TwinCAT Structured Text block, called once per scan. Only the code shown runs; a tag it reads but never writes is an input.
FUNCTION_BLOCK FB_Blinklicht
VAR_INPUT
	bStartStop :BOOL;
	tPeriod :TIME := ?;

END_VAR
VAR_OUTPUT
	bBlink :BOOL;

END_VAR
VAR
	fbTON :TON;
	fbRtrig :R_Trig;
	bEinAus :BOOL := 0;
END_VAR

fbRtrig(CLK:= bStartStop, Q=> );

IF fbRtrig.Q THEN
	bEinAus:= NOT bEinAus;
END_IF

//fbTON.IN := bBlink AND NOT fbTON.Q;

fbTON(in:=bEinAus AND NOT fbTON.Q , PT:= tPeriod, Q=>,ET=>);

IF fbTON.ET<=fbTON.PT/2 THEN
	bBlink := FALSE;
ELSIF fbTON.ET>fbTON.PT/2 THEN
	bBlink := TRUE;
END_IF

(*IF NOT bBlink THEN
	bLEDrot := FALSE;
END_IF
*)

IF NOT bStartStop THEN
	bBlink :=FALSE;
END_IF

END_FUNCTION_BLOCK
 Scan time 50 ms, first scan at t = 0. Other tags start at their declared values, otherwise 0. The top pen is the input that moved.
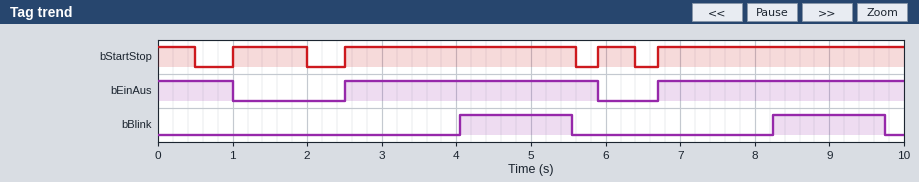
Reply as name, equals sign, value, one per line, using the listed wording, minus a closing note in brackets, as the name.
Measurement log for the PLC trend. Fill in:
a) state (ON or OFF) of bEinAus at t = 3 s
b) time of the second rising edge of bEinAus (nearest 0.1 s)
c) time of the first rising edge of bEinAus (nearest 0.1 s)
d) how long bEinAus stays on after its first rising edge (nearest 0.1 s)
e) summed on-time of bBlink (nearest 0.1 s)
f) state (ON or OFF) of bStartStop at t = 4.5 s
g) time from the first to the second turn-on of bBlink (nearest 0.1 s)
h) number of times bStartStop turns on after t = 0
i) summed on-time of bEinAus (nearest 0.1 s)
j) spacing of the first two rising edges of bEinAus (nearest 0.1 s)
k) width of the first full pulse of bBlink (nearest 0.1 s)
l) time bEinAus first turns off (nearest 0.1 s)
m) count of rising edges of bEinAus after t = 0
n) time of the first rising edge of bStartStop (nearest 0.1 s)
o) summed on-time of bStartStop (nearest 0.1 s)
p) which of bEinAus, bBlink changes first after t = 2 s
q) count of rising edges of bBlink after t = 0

state (ON or OFF) of bEinAus at t = 3 s = ON
time of the second rising edge of bEinAus = 6.7 s
time of the first rising edge of bEinAus = 2.5 s
how long bEinAus stays on after its first rising edge = 3.4 s
summed on-time of bBlink = 3.0 s
state (ON or OFF) of bStartStop at t = 4.5 s = ON
time from the first to the second turn-on of bBlink = 4.2 s
number of times bStartStop turns on after t = 0 = 4
summed on-time of bEinAus = 7.7 s
spacing of the first two rising edges of bEinAus = 4.2 s
width of the first full pulse of bBlink = 1.5 s
time bEinAus first turns off = 1.0 s
count of rising edges of bEinAus after t = 0 = 2
time of the first rising edge of bStartStop = 1.0 s
summed on-time of bStartStop = 8.4 s
which of bEinAus, bBlink changes first after t = 2 s = bEinAus
count of rising edges of bBlink after t = 0 = 2
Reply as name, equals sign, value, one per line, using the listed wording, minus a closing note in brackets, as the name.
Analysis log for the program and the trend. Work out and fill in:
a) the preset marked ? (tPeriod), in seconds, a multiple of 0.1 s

the preset marked ? (tPeriod), in seconds, a multiple of 0.1 s = 3.0 s
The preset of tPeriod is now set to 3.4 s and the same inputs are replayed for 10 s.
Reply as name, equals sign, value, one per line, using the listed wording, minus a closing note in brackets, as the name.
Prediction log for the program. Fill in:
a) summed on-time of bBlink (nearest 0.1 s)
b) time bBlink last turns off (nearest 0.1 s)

summed on-time of bBlink = 2.9 s
time bBlink last turns off = 5.6 s
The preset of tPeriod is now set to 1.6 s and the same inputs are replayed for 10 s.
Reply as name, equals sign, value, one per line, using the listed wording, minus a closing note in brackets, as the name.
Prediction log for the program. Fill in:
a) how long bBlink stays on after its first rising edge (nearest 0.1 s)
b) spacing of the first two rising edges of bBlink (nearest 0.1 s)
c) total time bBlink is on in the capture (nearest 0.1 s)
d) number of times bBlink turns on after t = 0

how long bBlink stays on after its first rising edge = 0.8 s
spacing of the first two rising edges of bBlink = 1.7 s
total time bBlink is on in the capture = 2.9 s
number of times bBlink turns on after t = 0 = 4
